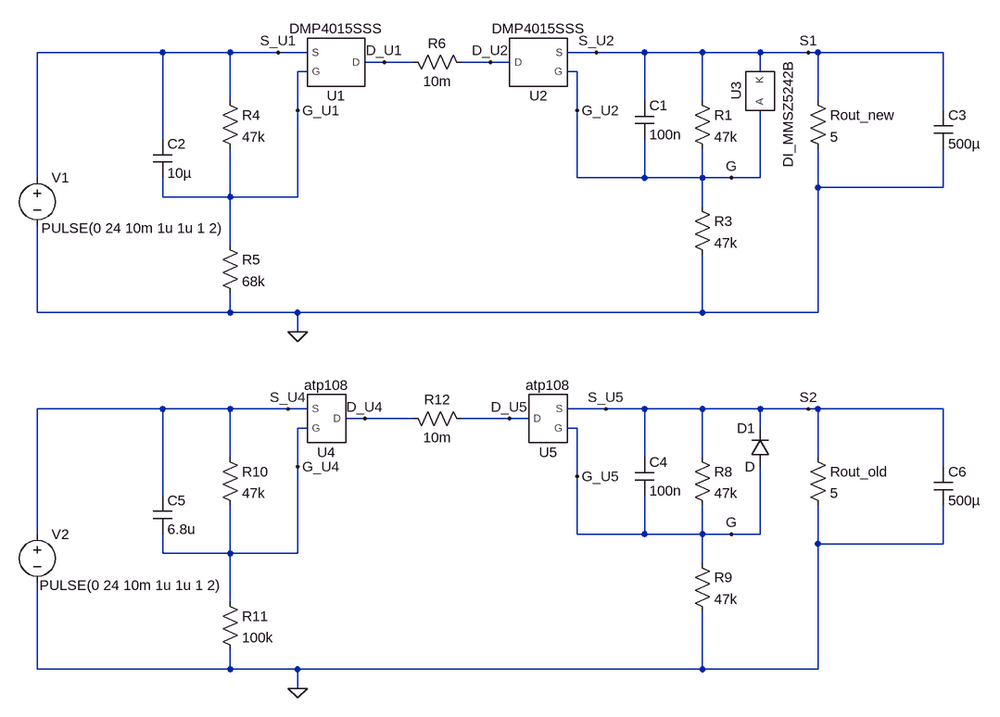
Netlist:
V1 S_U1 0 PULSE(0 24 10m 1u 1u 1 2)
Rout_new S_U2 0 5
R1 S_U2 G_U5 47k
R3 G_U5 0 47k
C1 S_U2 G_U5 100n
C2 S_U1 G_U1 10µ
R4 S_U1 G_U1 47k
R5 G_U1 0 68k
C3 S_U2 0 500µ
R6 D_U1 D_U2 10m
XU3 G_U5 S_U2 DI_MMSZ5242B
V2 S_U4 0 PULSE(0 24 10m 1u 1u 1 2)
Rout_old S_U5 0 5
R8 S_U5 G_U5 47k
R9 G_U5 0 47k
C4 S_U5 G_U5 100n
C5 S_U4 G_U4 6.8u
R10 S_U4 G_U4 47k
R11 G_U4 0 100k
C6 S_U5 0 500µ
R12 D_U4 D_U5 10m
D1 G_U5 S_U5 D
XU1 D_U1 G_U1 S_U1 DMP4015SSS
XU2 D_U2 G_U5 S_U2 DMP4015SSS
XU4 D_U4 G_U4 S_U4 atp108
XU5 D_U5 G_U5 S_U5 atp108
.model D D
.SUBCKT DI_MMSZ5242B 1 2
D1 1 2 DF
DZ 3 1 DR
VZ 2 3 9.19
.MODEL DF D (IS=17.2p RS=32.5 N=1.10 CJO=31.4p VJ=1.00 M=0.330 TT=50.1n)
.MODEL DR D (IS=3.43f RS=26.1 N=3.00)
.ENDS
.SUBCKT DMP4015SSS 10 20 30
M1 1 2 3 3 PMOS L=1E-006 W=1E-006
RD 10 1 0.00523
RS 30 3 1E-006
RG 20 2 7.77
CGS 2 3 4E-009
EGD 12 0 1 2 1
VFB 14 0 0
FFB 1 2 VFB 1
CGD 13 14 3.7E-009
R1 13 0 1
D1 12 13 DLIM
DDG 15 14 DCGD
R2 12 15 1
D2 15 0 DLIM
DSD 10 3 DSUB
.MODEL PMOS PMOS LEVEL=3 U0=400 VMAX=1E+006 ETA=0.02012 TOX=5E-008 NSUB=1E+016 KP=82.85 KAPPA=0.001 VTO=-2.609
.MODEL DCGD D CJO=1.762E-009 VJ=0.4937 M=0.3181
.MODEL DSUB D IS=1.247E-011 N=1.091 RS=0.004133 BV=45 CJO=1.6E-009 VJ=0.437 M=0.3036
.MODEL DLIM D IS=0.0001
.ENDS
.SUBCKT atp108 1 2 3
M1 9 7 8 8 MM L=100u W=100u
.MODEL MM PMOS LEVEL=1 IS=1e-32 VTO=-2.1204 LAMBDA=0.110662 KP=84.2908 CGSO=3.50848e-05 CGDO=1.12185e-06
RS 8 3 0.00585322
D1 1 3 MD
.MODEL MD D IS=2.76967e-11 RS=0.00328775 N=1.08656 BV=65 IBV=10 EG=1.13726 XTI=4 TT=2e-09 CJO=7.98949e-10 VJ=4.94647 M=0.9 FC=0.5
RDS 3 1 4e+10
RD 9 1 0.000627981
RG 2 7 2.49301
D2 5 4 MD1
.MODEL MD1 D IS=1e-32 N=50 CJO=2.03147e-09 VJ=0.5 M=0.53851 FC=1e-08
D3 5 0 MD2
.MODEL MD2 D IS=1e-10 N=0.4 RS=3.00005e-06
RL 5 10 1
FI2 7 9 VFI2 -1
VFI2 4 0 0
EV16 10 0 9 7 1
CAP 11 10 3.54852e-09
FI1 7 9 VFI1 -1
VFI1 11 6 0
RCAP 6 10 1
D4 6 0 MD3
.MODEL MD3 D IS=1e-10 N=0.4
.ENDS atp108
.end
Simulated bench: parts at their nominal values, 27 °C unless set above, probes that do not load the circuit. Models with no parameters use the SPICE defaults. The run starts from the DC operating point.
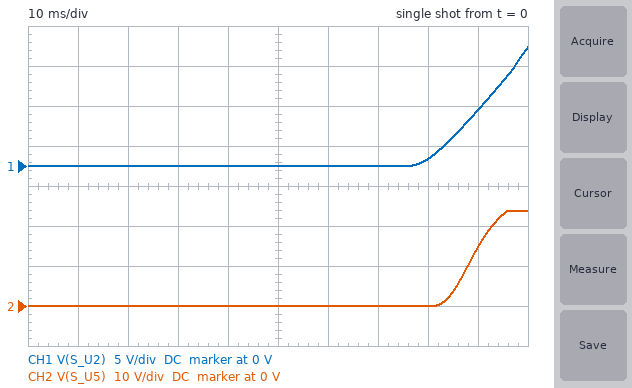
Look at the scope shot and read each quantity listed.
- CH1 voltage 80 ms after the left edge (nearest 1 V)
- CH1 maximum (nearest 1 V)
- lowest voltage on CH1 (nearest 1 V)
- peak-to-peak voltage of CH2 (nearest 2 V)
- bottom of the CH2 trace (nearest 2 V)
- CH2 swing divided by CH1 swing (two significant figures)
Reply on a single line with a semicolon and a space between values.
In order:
1 V; 15 V; 0 V; 24 V; 0 V; 1.6
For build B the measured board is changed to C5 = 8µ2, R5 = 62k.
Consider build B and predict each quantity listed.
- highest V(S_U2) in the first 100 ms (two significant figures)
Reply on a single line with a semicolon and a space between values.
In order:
22 V
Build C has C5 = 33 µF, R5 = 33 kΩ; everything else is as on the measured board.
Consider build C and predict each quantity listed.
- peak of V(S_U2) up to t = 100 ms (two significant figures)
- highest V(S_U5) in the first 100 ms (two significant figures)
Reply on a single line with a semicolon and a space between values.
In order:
24 V; 1.8 V
